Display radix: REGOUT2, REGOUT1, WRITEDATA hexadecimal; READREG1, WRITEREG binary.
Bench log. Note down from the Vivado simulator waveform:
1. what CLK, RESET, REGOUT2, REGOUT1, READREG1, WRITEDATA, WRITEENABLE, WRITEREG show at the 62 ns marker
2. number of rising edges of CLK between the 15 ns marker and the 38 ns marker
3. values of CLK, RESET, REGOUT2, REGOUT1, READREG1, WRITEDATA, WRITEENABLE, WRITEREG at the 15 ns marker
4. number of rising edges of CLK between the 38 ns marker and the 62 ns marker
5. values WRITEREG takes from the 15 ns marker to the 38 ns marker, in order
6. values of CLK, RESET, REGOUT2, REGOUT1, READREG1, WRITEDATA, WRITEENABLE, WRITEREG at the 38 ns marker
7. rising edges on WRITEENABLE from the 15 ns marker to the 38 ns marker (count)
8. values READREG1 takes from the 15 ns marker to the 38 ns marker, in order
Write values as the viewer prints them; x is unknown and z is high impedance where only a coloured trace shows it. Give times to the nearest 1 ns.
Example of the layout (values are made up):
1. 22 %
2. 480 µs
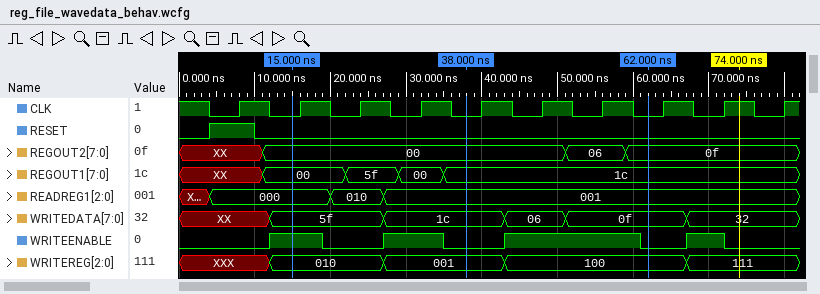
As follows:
1. CLK=0, RESET=0, REGOUT2=0f, REGOUT1=1c, READREG1=001, WRITEDATA=0f, WRITEENABLE=0, WRITEREG=100
2. 3
3. CLK=0, RESET=0, REGOUT2=00, REGOUT1=00, READREG1=000, WRITEDATA=5f, WRITEENABLE=1, WRITEREG=010
4. 3
5. 010, 001
6. CLK=0, RESET=0, REGOUT2=00, REGOUT1=1c, READREG1=001, WRITEDATA=1c, WRITEENABLE=0, WRITEREG=001
7. 1
8. 000, 010, 001
